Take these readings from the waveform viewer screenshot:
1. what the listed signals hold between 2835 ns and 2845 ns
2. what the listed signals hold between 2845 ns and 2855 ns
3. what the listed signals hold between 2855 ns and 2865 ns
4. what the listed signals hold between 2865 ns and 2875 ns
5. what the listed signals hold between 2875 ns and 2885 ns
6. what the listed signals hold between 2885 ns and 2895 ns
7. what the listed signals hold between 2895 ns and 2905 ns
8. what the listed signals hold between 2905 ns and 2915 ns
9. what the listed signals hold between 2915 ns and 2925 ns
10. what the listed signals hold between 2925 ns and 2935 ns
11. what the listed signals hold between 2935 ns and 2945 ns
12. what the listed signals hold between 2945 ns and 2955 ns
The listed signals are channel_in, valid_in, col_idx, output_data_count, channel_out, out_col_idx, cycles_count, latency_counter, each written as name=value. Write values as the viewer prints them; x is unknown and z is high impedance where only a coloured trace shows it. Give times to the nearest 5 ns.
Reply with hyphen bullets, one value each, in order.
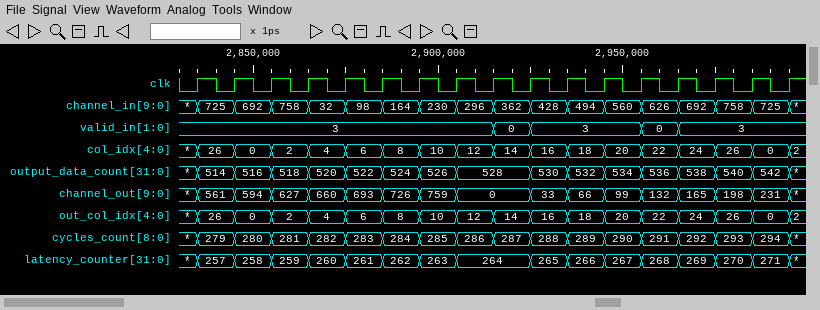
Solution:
- channel_in=725, valid_in=3, col_idx=26, output_data_count=514, channel_out=561, out_col_idx=26, cycles_count=279, latency_counter=257
- channel_in=692, valid_in=3, col_idx=0, output_data_count=516, channel_out=594, out_col_idx=0, cycles_count=280, latency_counter=258
- channel_in=758, valid_in=3, col_idx=2, output_data_count=518, channel_out=627, out_col_idx=2, cycles_count=281, latency_counter=259
- channel_in=32, valid_in=3, col_idx=4, output_data_count=520, channel_out=660, out_col_idx=4, cycles_count=282, latency_counter=260
- channel_in=98, valid_in=3, col_idx=6, output_data_count=522, channel_out=693, out_col_idx=6, cycles_count=283, latency_counter=261
- channel_in=164, valid_in=3, col_idx=8, output_data_count=524, channel_out=726, out_col_idx=8, cycles_count=284, latency_counter=262
- channel_in=230, valid_in=3, col_idx=10, output_data_count=526, channel_out=759, out_col_idx=10, cycles_count=285, latency_counter=263
- channel_in=296, valid_in=3, col_idx=12, output_data_count=528, channel_out=0, out_col_idx=12, cycles_count=286, latency_counter=264
- channel_in=362, valid_in=0, col_idx=14, output_data_count=528, channel_out=0, out_col_idx=14, cycles_count=287, latency_counter=264
- channel_in=428, valid_in=3, col_idx=16, output_data_count=530, channel_out=33, out_col_idx=16, cycles_count=288, latency_counter=265
- channel_in=494, valid_in=3, col_idx=18, output_data_count=532, channel_out=66, out_col_idx=18, cycles_count=289, latency_counter=266
- channel_in=560, valid_in=3, col_idx=20, output_data_count=534, channel_out=99, out_col_idx=20, cycles_count=290, latency_counter=267
